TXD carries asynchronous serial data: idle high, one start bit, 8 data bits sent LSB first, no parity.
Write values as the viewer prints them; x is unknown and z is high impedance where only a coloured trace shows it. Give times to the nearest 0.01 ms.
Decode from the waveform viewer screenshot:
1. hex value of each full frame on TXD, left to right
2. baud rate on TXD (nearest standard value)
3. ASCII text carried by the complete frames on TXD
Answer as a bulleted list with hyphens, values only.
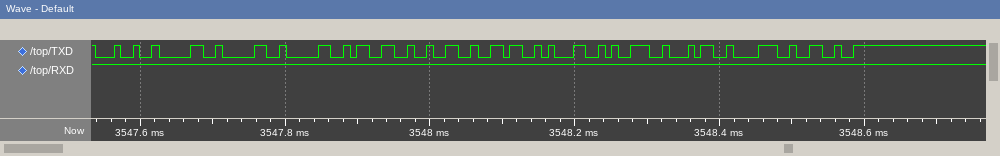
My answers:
- 24, 30, 30, 30, 33, 32, 36, 31, 39, 34, 38, 26
- 115200 baud
- "$0003261948&"
